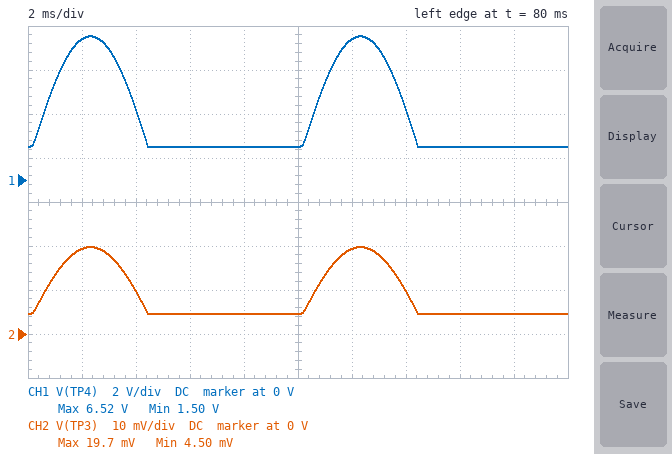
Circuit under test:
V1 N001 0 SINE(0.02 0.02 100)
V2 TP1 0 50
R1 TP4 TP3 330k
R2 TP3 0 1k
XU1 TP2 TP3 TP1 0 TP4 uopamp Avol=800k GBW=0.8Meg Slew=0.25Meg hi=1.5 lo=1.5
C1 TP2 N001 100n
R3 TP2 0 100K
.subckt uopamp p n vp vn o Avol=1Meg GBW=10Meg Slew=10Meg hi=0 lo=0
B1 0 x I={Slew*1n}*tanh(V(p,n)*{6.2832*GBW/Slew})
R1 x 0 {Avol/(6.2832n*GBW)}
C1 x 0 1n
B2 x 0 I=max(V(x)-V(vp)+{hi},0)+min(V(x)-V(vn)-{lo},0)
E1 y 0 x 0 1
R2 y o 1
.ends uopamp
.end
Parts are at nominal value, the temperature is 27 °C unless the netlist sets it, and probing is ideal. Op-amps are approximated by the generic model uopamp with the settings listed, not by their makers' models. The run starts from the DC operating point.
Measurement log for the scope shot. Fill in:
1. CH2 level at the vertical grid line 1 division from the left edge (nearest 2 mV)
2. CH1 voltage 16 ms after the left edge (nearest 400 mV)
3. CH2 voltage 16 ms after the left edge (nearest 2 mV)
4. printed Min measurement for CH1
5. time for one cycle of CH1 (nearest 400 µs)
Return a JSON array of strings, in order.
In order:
["20 mV", "1.6 V", "4 mV", "1.50 V", "10.0 ms"]
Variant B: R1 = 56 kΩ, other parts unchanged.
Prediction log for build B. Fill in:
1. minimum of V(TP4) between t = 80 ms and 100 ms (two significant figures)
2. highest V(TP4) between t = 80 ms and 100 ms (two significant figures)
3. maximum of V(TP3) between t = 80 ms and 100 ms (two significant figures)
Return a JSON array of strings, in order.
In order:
["1.5 V", "1.5 V", "26 mV"]
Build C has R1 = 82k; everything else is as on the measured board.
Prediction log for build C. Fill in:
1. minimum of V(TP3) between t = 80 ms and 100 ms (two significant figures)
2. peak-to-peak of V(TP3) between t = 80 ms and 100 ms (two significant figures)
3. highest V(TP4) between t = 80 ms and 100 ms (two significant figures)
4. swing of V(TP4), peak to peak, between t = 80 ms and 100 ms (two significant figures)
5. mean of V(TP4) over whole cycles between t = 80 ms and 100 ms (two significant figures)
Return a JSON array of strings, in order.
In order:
["18 mV", "1.7 mV", "1.6 V", "140 mV", "1.5 V"]
